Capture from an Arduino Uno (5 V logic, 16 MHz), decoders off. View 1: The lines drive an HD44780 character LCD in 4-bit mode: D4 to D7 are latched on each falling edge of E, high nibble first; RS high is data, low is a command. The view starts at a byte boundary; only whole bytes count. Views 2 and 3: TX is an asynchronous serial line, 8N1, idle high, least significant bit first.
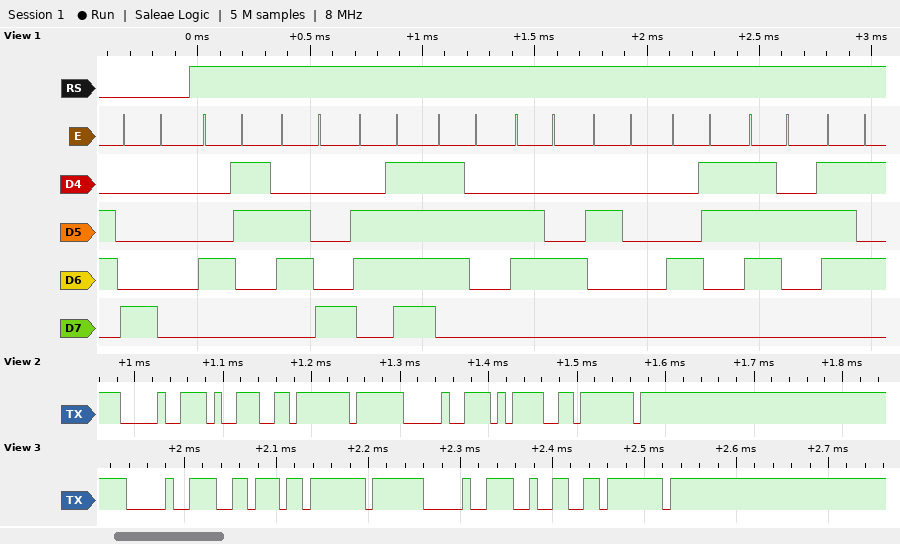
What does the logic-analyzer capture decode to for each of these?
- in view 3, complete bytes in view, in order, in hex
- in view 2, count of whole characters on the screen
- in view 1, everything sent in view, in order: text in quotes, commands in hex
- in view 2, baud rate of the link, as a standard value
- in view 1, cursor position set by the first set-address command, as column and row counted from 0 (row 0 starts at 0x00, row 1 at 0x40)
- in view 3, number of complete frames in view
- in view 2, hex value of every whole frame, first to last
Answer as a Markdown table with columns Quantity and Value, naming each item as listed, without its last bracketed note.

| Quantity | Value |
|---|---|
| in view 3, complete bytes in view, in order, in hex | 0x90 0x76 0x7F 0x90 0x32 0x7F |
| in view 2, count of whole characters on the screen | 6 |
| in view 1, everything sent in view, in order: text in quotes, commands in hex | 0x80 "Chord Cru" |
| in view 2, baud rate of the link, as a standard value | 115200 baud |
| in view 1, cursor position set by the first set-address command, as column and row counted from 0 | column 0, row 0 |
| in view 3, number of complete frames in view | 6 |
| in view 2, hex value of every whole frame, first to last | 90 39 7F 90 3D 7F |
